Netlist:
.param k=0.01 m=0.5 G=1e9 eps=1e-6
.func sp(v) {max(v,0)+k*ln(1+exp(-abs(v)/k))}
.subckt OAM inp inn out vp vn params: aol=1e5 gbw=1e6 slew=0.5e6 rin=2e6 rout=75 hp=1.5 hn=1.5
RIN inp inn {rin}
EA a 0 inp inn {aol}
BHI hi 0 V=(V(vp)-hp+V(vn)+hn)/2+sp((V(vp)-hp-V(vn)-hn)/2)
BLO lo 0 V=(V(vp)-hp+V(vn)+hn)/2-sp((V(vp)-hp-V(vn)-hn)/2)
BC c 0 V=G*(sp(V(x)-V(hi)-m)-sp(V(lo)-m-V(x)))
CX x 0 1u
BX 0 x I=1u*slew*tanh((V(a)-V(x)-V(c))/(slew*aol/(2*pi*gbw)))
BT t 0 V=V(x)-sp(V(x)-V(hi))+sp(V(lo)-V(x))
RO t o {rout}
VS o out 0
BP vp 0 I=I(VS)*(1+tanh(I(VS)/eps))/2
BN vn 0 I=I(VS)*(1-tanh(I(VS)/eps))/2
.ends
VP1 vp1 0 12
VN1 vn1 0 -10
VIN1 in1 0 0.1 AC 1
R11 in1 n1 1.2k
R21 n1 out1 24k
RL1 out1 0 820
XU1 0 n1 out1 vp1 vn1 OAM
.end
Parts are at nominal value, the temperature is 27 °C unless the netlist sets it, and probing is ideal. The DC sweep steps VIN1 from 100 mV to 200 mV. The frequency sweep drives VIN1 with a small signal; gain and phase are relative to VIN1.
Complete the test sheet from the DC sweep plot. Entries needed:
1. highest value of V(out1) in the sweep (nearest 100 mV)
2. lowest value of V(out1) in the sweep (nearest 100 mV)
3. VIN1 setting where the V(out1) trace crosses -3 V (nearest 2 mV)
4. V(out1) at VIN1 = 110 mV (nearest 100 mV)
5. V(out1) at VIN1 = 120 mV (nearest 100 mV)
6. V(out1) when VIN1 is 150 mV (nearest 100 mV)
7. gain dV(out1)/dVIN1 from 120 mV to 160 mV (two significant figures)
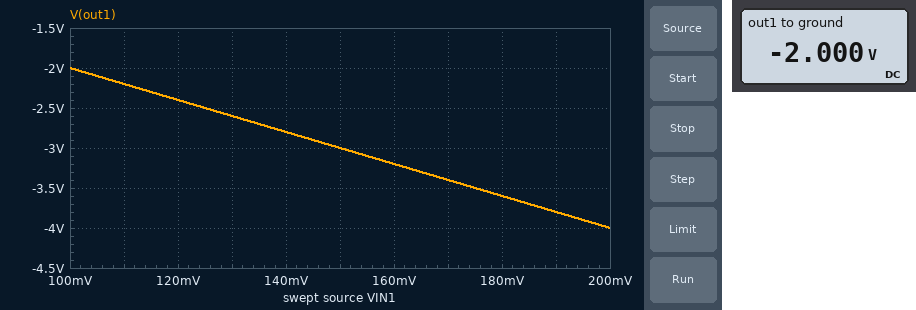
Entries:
-2.0 V
-4.0 V
150 mV
-2.2 V
-2.4 V
-3.0 V
-20 V/V
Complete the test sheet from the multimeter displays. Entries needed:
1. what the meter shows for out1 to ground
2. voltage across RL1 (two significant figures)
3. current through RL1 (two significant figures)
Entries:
-2.000 V
2.0 V
2.4 mA
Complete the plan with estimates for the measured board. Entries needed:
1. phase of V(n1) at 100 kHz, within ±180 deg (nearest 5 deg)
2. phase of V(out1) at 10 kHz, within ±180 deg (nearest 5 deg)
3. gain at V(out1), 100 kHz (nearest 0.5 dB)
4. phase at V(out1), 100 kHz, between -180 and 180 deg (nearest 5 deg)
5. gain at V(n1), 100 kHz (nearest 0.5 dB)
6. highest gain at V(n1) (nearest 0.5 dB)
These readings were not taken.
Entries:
25 deg
165 deg
18.0 dB
115 deg
-1.0 dB
-0.5 dB
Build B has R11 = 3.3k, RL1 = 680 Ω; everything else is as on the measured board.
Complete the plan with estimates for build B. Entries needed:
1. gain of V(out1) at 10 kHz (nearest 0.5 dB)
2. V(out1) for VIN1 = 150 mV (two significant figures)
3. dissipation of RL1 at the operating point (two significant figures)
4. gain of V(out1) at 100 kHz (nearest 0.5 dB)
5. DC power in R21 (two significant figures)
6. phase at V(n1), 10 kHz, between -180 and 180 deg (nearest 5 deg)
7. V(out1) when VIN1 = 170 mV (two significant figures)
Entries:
17.0 dB
-1.1 V
780 µW
14.5 dB
22 µW
85 deg
-1.2 V
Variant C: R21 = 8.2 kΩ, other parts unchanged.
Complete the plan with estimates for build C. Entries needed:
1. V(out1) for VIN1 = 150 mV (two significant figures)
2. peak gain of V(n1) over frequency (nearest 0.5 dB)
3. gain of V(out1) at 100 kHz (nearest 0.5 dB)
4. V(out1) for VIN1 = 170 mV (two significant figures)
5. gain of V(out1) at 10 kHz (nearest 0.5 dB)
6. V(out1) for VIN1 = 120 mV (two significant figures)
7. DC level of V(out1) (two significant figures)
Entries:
-1.0 V
-1.0 dB
14.5 dB
-1.2 V
16.5 dB
-820 mV
-680 mV
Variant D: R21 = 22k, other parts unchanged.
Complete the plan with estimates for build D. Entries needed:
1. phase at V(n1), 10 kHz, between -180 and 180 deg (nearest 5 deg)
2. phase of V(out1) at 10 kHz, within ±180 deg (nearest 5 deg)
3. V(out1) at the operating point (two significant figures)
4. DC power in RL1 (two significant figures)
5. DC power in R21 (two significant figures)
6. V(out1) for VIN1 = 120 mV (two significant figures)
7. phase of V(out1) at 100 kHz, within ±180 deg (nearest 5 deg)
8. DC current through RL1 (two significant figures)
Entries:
80 deg
170 deg
-1.8 V
4.1 mW
150 µW
-2.2 V
115 deg
2.2 mA
